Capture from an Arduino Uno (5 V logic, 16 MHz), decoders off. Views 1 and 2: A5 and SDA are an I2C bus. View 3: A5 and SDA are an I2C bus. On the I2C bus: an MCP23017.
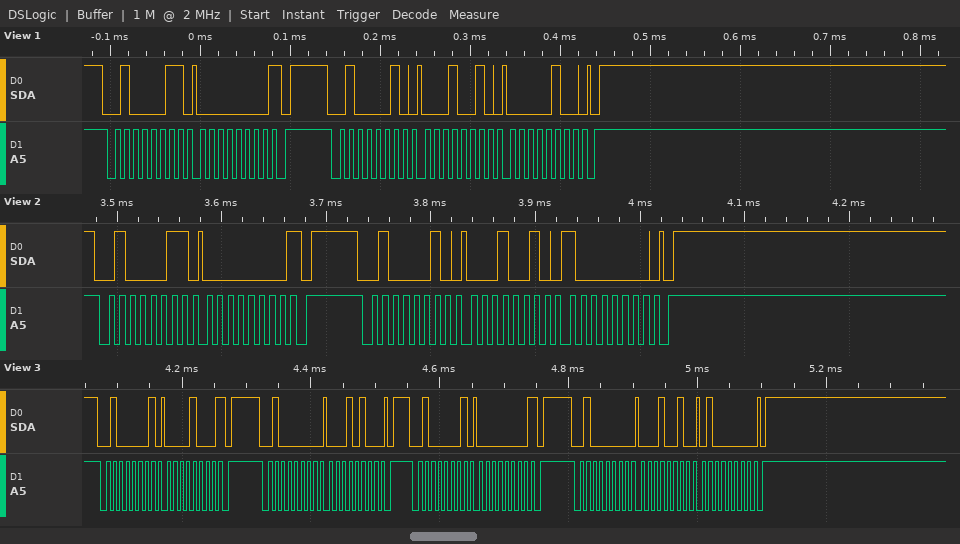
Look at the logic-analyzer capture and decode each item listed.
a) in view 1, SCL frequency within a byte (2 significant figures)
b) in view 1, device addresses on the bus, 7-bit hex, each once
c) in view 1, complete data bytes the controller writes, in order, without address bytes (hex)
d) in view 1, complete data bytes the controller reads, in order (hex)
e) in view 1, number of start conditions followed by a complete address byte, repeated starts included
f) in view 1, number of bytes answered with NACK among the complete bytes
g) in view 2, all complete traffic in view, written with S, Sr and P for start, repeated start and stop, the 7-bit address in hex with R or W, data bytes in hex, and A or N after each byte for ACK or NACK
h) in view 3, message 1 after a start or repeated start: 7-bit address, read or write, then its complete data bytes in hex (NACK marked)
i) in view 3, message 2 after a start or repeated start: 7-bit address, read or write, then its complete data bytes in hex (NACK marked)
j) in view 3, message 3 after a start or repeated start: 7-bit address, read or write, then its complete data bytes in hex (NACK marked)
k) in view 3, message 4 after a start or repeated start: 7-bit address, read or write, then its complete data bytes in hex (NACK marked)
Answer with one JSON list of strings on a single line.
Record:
["100 kHz", "0x21", "12 04", "00", "2", "1", "S 21R A 00 N P S 21W A 12 A 80 A P", "0x20 read: 08 NACK", "0x20 write: 14", "0x20 read: 00 NACK", "0x20 write: 12 40"]
